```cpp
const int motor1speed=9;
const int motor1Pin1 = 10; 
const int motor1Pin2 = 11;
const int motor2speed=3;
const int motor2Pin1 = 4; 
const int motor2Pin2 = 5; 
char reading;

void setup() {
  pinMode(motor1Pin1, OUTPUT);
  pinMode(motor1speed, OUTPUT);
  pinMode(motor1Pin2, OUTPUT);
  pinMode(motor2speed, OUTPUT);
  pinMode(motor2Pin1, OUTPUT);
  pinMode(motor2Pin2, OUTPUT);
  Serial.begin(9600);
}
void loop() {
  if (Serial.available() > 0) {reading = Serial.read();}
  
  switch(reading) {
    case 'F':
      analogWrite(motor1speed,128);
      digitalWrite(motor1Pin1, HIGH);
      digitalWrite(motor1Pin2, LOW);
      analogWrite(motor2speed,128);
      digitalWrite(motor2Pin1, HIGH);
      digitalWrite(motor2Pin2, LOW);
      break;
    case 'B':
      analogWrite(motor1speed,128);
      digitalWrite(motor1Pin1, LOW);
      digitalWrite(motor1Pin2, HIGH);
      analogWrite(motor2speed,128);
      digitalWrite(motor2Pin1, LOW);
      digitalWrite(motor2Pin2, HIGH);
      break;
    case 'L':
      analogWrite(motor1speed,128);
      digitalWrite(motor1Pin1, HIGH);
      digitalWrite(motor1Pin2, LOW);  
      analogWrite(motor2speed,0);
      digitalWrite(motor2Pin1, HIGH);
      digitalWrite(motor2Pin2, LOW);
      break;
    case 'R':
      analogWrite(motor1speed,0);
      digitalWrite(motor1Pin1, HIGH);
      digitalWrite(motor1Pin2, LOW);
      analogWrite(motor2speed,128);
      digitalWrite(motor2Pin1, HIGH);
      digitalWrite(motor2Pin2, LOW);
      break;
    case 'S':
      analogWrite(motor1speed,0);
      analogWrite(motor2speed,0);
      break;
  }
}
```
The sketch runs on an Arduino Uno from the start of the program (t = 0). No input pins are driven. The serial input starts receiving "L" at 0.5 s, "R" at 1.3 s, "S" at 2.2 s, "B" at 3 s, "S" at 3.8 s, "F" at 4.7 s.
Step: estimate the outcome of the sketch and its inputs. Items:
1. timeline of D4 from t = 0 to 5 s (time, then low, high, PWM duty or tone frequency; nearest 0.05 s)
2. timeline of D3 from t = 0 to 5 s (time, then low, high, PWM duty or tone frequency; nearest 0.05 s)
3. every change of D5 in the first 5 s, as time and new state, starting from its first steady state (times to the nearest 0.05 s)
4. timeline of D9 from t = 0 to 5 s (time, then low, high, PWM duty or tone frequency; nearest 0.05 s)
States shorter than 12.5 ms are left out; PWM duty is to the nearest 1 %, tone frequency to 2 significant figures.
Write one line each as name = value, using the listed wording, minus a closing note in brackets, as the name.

timeline of D4 from t = 0 to 5 s = 0 s low; 0.5 s high; 3 s low; 4.7 s high
timeline of D3 from t = 0 to 5 s = 0 s low; 1.3 s PWM 50 %; 2.2 s low; 3 s PWM 50 %; 3.8 s low; 4.7 s PWM 50 %
every change of D5 in the first 5 s, as time and new state, starting from its first steady state = 0 s low; 3 s high; 4.7 s low
timeline of D9 from t = 0 to 5 s = 0 s low; 0.5 s PWM 50 %; 1.3 s low; 3 s PWM 50 %; 3.8 s low; 4.7 s PWM 50 %
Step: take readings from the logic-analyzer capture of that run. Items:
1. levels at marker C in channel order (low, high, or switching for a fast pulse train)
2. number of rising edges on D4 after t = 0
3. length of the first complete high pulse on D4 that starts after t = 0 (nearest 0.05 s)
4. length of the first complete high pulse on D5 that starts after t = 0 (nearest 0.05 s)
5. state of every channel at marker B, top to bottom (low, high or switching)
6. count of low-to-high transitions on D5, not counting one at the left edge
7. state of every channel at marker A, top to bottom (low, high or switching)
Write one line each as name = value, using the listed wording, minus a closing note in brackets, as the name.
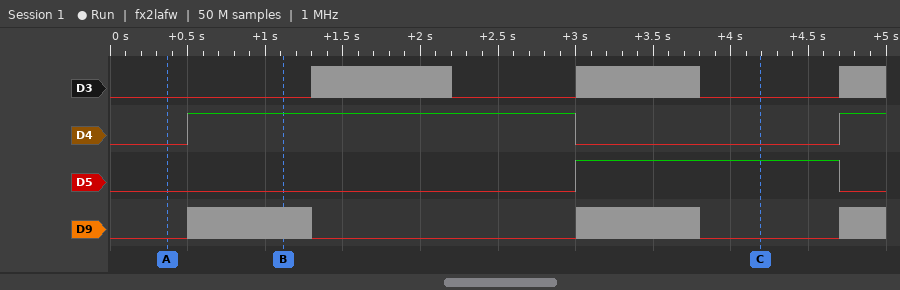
levels at marker C in channel order = D3 low, D4 low, D5 high, D9 low
number of rising edges on D4 after t = 0 = 2
length of the first complete high pulse on D4 that starts after t = 0 = 2.50 s
length of the first complete high pulse on D5 that starts after t = 0 = 1.70 s
state of every channel at marker B, top to bottom = D3 low, D4 high, D5 low, D9 switching
count of low-to-high transitions on D5, not counting one at the left edge = 1
state of every channel at marker A, top to bottom = D3 low, D4 low, D5 low, D9 low
